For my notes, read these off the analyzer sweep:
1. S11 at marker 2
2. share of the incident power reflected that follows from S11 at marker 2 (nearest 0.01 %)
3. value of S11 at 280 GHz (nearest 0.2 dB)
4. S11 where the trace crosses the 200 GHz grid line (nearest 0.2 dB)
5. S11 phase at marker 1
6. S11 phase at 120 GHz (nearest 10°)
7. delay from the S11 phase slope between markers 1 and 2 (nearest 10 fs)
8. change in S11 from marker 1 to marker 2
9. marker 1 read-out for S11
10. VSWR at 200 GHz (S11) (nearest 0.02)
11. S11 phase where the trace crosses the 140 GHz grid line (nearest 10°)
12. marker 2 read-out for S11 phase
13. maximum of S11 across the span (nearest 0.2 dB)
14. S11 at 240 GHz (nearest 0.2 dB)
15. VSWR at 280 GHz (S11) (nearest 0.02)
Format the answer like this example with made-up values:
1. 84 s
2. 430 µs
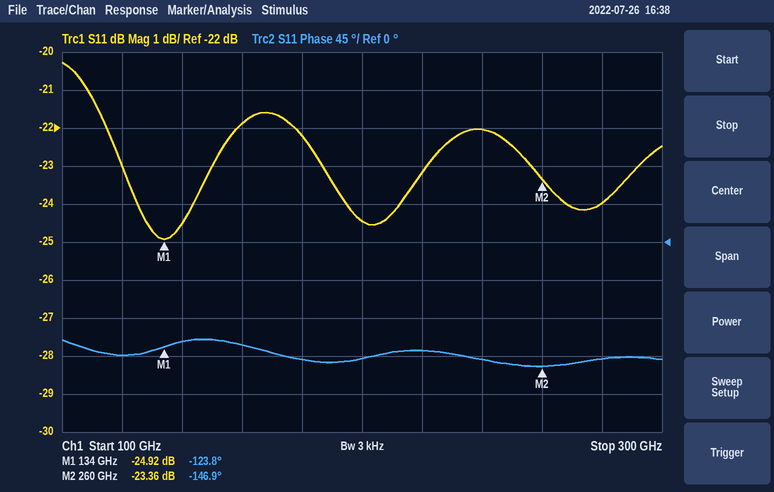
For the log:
1. -23.36 dB
2. 0.46 %
3. -24.0 dB
4. -24.4 dB
5. -123.8°
6. -130°
7. 510 fs
8. 1.56 dB
9. -24.92 dB
10. 1.12
11. -120°
12. -146.9°
13. -20.2 dB
14. -22.0 dB
15. 1.14
